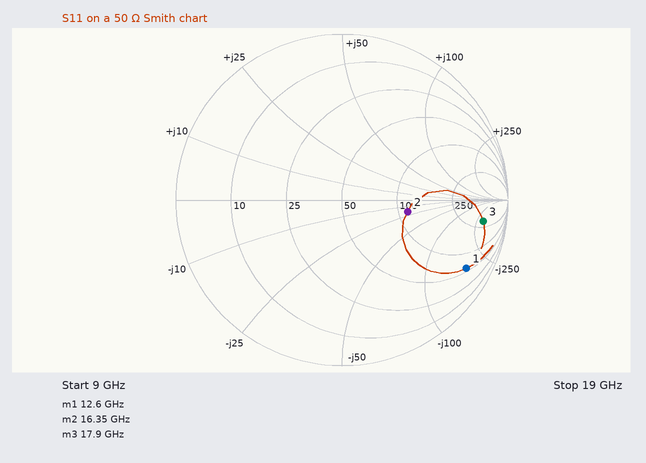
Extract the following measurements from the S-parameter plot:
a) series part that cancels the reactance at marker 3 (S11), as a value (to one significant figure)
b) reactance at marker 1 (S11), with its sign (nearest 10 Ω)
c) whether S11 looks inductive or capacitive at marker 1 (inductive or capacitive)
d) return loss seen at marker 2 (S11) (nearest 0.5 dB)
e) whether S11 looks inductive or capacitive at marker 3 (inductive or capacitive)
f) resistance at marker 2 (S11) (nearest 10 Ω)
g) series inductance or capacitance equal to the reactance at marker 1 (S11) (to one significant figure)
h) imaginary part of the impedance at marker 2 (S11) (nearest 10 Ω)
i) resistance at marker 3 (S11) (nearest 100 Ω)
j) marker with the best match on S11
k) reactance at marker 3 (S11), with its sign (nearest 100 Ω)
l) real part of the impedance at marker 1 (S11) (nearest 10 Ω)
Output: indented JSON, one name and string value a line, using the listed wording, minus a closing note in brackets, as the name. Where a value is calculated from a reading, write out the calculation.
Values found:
{
  "series part that cancels the reactance at marker 3 (S11), as a value": "L = 300 Ω/(2π × 17.9 GHz) ≈ 3 nH",
  "reactance at marker 1 (S11), with its sign": "-180 Ω",
  "whether S11 looks inductive or capacitive at marker 1": "capacitive",
  "return loss seen at marker 2 (S11)": "8.0 dB",
  "whether S11 looks inductive or capacitive at marker 3": "capacitive",
  "resistance at marker 2 (S11)": "110 Ω",
  "series inductance or capacitance equal to the reactance at marker 1 (S11)": "C = 1/(2π × 12.6 GHz × 180 Ω) ≈ 70 fF",
  "imaginary part of the impedance at marker 2 (S11)": "-20 Ω",
  "resistance at marker 3 (S11)": "300 Ω",
  "marker with the best match on S11": "marker 2",
  "reactance at marker 3 (S11), with its sign": "-300 Ω",
  "real part of the impedance at marker 1 (S11)": "60 Ω"
}
